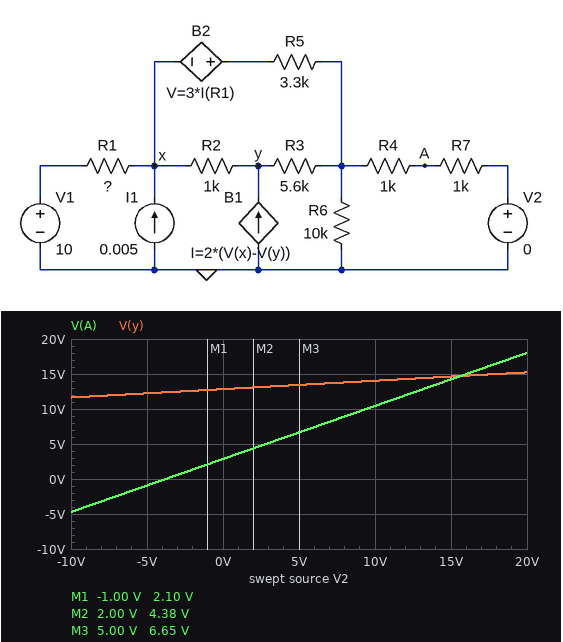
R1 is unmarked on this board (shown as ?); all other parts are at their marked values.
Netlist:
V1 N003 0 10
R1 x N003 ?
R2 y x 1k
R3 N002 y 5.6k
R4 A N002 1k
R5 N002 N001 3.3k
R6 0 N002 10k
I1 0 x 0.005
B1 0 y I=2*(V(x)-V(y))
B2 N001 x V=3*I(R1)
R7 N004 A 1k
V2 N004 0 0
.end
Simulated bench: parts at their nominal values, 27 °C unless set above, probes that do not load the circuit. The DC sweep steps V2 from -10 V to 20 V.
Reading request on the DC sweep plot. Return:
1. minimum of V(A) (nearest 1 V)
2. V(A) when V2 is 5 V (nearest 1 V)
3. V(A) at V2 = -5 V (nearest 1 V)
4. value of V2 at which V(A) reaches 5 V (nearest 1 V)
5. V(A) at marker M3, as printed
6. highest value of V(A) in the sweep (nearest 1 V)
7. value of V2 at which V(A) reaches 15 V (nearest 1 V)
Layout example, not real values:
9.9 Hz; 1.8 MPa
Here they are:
-5 V; 7 V; -1 V; 3 V; 6.65 V; 18 V; 16 V
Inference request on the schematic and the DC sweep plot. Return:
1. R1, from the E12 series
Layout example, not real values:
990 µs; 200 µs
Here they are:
1 kΩ
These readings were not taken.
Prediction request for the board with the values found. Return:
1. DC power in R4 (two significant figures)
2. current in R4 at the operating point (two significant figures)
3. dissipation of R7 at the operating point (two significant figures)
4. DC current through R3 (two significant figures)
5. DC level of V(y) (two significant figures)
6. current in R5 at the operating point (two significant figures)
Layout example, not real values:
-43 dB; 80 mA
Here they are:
8.2 mW; 2.9 mA; 8.2 mW; 1.3 mA; 13 V; 2.2 mA
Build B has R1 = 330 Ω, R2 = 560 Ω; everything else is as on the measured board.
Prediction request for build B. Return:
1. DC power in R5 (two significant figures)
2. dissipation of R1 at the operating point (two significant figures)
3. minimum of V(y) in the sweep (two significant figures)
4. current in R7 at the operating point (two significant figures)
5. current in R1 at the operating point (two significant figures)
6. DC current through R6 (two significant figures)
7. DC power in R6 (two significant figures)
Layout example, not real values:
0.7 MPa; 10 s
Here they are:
11 mW; 3.3 mW; 11 V; 2.5 mA; 3.1 mA; 490 µA; 2.4 mW
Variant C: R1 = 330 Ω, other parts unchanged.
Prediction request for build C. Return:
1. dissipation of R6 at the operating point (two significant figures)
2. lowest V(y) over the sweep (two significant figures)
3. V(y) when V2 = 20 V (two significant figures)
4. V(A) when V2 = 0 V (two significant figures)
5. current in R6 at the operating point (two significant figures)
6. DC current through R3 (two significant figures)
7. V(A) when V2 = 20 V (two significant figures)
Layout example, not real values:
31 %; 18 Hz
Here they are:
2.4 mW; 11 V; 12 V; 2.5 V; 490 µA; 1.1 mA; 17 V
